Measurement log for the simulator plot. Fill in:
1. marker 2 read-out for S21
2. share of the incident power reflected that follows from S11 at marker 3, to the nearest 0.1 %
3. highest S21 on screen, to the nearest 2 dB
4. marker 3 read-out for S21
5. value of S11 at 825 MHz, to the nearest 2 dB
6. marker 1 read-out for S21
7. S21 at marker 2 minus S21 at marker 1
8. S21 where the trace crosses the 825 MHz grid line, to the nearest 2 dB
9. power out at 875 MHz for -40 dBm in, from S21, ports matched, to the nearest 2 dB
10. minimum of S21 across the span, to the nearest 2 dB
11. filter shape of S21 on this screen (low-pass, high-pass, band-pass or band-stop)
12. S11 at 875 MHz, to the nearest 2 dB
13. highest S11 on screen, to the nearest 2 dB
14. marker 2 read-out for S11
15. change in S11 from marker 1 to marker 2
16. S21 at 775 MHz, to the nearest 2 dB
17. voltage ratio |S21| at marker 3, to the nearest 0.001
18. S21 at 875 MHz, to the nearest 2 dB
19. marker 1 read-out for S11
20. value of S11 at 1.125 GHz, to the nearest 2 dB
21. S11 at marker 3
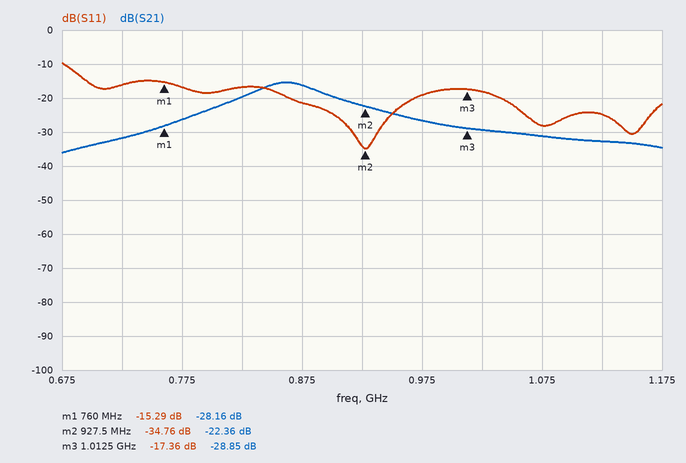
-22.36 dB
1.8 %
-16 dB
-28.85 dB
-16 dB
-28.16 dB
5.80 dB
-20 dB
-56 dBm
-36 dB
band-pass
-22 dB
-10 dB
-34.76 dB
-19.47 dB
-26 dB
0.036
-16 dB
-15.29 dB
-24 dB
-17.36 dB
